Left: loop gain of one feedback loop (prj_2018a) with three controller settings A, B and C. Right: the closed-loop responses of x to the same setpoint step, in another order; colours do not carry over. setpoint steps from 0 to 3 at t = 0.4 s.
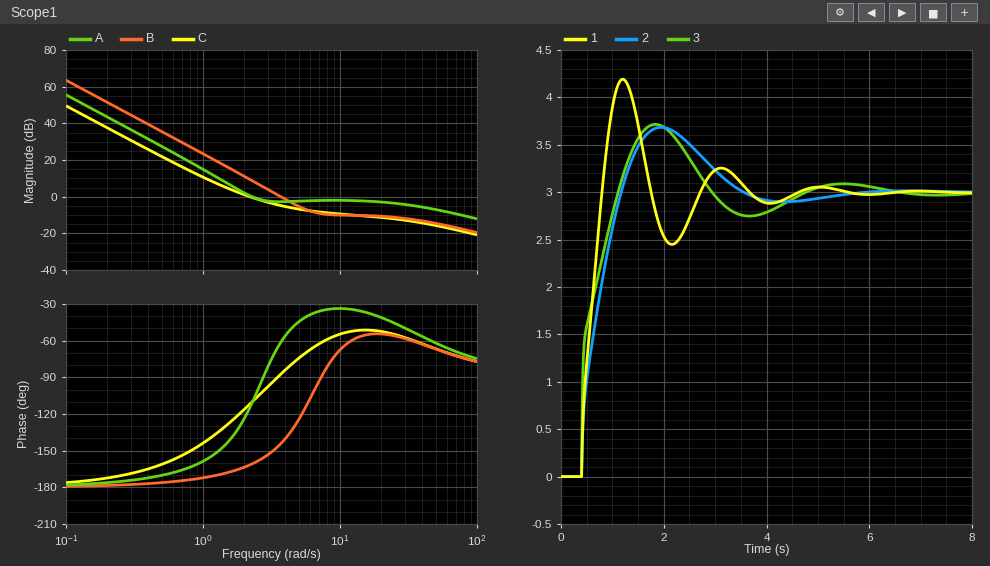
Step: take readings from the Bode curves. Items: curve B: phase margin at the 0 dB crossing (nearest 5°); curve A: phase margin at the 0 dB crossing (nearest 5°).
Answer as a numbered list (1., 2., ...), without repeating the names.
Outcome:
1. 35°
2. 70°
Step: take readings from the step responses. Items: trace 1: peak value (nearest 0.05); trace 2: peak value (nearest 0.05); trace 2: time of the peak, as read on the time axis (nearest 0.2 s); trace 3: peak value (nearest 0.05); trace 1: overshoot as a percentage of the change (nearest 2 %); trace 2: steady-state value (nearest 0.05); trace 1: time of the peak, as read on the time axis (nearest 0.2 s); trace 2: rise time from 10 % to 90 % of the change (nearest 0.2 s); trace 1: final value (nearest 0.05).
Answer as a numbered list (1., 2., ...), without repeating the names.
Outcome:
1. 4.20
2. 3.70
3. 2.0 s
4. 3.70
5. 40 %
6. 3.00
7. 1.2 s
8. 0.6 s
9. 3.00
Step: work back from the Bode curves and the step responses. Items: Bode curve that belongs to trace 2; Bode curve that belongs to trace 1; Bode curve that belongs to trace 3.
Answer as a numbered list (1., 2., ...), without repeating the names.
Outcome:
1. C
2. B
3. A
